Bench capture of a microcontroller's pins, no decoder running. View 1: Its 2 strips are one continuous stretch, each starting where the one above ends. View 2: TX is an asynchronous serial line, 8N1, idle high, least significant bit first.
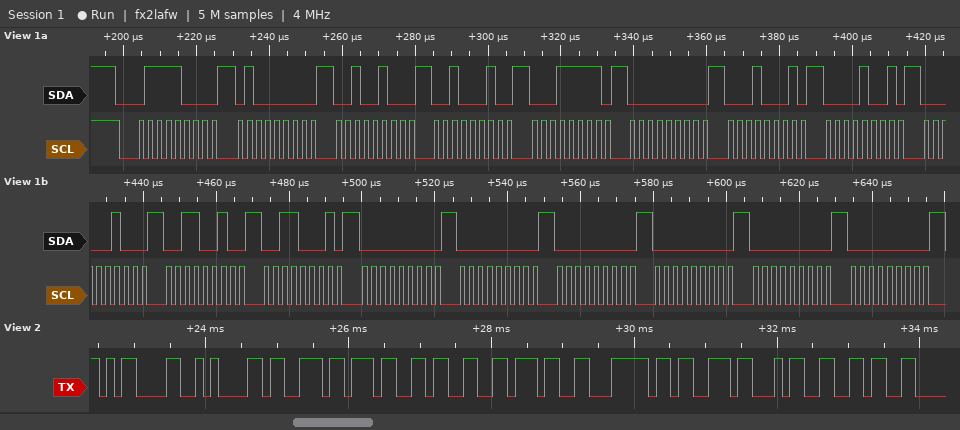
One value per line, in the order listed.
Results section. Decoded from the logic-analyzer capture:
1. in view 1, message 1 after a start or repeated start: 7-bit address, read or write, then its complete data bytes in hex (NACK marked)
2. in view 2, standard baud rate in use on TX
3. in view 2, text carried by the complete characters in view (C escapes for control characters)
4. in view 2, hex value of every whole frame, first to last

0x3C write: 40 24 22 1F 00 11 09 04 32 31 00 00 00 00 00 00
9600 baud
"\r\ns737|s46"
0D 0A 73 37 33 37 7C 73 34 36
